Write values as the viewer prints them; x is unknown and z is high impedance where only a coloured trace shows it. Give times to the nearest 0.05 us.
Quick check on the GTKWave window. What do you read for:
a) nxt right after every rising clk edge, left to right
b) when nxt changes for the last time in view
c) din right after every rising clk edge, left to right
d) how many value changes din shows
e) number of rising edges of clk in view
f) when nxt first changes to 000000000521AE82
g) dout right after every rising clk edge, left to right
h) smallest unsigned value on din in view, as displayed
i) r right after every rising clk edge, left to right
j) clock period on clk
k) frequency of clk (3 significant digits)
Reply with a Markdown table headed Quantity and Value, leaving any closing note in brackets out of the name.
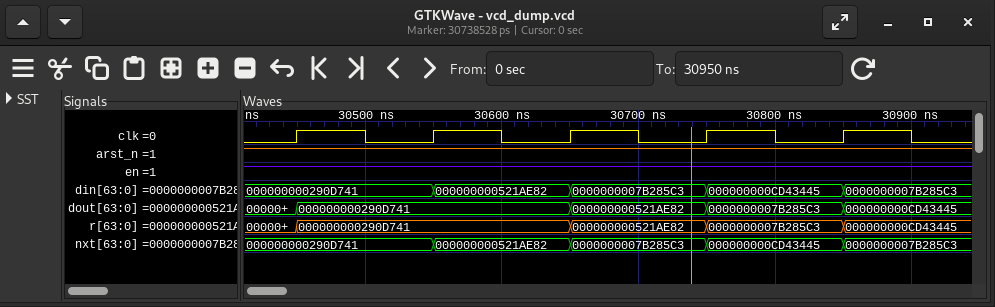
| Quantity | Value |
|---|---|
| nxt right after every rising clk edge, left to right | 000000000290D741, 000000000521AE82, 0000000007B285C3, 000000000CD43445, 0000000007B285C3 |
| when nxt changes for the last time in view | 30.85 us |
| din right after every rising clk edge, left to right | 000000000290D741, 000000000521AE82, 0000000007B285C3, 000000000CD43445, 0000000007B285C3 |
| how many value changes din shows | 4 |
| number of rising edges of clk in view | 5 |
| when nxt first changes to 000000000521AE82 | 30.55 us |
| dout right after every rising clk edge, left to right | 000000000290D741, 000000000290D741, 000000000521AE82, 0000000007B285C3, 000000000CD43445 |
| smallest unsigned value on din in view, as displayed | 000000000290D741 |
| r right after every rising clk edge, left to right | 000000000290D741, 000000000290D741, 000000000521AE82, 0000000007B285C3, 000000000CD43445 |
| clock period on clk | 0.1 us |
| frequency of clk | 10.0 MHz |
